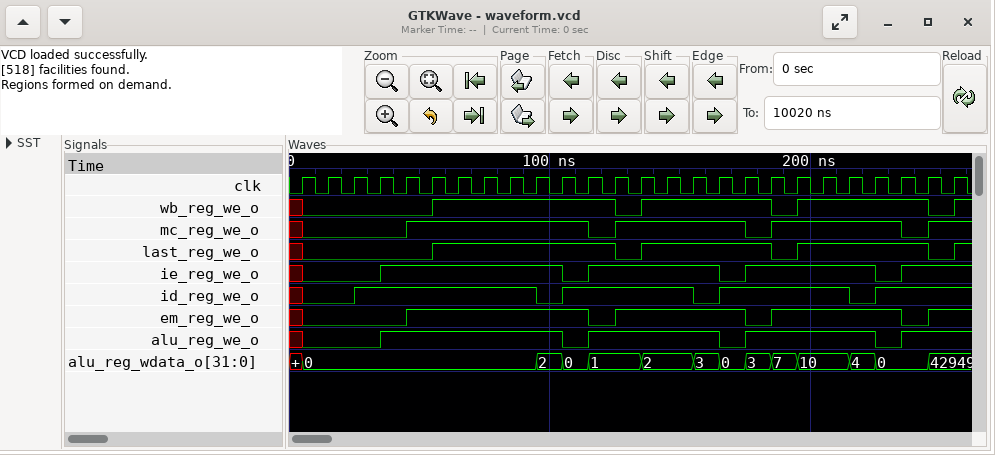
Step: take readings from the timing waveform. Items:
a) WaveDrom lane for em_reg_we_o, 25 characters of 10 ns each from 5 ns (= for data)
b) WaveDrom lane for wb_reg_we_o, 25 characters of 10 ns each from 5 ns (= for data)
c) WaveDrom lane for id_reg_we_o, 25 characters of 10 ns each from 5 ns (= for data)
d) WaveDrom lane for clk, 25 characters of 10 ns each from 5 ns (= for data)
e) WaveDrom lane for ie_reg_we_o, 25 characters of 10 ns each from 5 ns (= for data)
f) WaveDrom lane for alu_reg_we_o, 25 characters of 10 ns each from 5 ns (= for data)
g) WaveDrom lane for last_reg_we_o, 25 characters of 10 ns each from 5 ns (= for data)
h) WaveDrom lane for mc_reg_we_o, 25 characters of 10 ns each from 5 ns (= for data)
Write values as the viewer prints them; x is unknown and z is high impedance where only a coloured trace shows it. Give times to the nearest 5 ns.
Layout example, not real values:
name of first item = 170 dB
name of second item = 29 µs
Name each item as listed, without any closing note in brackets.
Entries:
WaveDrom lane for em_reg_we_o, 25 characters of 10 ns each from 5 ns = {name: 'em_reg_we_o', wave: '0...1......01....01....01'}
WaveDrom lane for wb_reg_we_o, 25 characters of 10 ns each from 5 ns = {name: 'wb_reg_we_o', wave: '0....1......01....01....0'}
WaveDrom lane for id_reg_we_o, 25 characters of 10 ns each from 5 ns = {name: 'id_reg_we_o', wave: '0.1......01....01....01..'}
WaveDrom lane for clk, 25 characters of 10 ns each from 5 ns = {name: 'clk', wave: 'p........................'}
WaveDrom lane for ie_reg_we_o, 25 characters of 10 ns each from 5 ns = {name: 'ie_reg_we_o', wave: '0..1......01....01....01.'}
WaveDrom lane for alu_reg_we_o, 25 characters of 10 ns each from 5 ns = {name: 'alu_reg_we_o', wave: '0..1......01....01....01.'}
WaveDrom lane for last_reg_we_o, 25 characters of 10 ns each from 5 ns = {name: 'last_reg_we_o', wave: '0....1......01....01....0'}
WaveDrom lane for mc_reg_we_o, 25 characters of 10 ns each from 5 ns = {name: 'mc_reg_we_o', wave: '0...1......01....01....01'}
